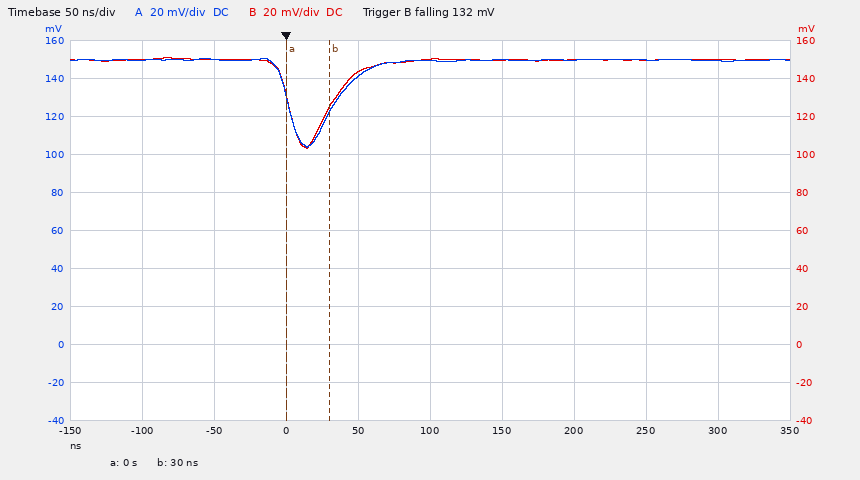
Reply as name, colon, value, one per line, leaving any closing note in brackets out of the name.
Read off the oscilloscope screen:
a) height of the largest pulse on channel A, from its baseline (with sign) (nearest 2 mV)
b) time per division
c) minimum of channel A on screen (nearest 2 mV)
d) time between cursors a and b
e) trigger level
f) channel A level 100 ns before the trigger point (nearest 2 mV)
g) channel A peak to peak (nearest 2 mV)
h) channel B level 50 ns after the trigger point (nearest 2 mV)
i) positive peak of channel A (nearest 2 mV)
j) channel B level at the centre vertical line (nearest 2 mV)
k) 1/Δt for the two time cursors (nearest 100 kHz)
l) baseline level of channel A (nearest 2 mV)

height of the largest pulse on channel A, from its baseline (with sign): -46 mV
time per division: 50 ns
minimum of channel A on screen: 104 mV
time between cursors a and b: 30 ns
trigger level: 132 mV
channel A level 100 ns before the trigger point: 150 mV
channel A peak to peak: 46 mV
channel B level 50 ns after the trigger point: 144 mV
positive peak of channel A: 150 mV
channel B level at the centre vertical line: 150 mV
1/Δt for the two time cursors: 33.3 MHz
baseline level of channel A: 150 mV
